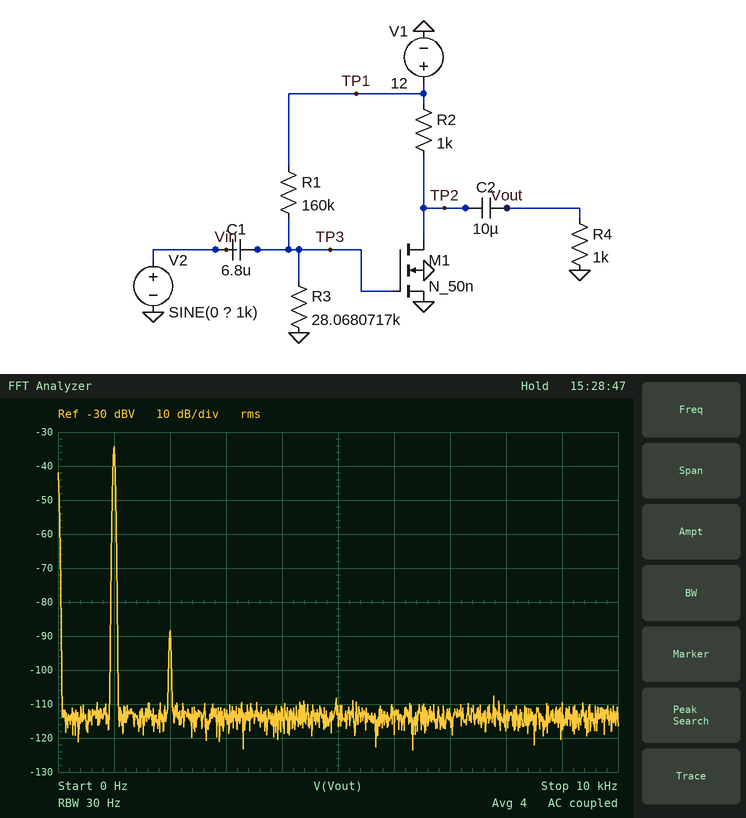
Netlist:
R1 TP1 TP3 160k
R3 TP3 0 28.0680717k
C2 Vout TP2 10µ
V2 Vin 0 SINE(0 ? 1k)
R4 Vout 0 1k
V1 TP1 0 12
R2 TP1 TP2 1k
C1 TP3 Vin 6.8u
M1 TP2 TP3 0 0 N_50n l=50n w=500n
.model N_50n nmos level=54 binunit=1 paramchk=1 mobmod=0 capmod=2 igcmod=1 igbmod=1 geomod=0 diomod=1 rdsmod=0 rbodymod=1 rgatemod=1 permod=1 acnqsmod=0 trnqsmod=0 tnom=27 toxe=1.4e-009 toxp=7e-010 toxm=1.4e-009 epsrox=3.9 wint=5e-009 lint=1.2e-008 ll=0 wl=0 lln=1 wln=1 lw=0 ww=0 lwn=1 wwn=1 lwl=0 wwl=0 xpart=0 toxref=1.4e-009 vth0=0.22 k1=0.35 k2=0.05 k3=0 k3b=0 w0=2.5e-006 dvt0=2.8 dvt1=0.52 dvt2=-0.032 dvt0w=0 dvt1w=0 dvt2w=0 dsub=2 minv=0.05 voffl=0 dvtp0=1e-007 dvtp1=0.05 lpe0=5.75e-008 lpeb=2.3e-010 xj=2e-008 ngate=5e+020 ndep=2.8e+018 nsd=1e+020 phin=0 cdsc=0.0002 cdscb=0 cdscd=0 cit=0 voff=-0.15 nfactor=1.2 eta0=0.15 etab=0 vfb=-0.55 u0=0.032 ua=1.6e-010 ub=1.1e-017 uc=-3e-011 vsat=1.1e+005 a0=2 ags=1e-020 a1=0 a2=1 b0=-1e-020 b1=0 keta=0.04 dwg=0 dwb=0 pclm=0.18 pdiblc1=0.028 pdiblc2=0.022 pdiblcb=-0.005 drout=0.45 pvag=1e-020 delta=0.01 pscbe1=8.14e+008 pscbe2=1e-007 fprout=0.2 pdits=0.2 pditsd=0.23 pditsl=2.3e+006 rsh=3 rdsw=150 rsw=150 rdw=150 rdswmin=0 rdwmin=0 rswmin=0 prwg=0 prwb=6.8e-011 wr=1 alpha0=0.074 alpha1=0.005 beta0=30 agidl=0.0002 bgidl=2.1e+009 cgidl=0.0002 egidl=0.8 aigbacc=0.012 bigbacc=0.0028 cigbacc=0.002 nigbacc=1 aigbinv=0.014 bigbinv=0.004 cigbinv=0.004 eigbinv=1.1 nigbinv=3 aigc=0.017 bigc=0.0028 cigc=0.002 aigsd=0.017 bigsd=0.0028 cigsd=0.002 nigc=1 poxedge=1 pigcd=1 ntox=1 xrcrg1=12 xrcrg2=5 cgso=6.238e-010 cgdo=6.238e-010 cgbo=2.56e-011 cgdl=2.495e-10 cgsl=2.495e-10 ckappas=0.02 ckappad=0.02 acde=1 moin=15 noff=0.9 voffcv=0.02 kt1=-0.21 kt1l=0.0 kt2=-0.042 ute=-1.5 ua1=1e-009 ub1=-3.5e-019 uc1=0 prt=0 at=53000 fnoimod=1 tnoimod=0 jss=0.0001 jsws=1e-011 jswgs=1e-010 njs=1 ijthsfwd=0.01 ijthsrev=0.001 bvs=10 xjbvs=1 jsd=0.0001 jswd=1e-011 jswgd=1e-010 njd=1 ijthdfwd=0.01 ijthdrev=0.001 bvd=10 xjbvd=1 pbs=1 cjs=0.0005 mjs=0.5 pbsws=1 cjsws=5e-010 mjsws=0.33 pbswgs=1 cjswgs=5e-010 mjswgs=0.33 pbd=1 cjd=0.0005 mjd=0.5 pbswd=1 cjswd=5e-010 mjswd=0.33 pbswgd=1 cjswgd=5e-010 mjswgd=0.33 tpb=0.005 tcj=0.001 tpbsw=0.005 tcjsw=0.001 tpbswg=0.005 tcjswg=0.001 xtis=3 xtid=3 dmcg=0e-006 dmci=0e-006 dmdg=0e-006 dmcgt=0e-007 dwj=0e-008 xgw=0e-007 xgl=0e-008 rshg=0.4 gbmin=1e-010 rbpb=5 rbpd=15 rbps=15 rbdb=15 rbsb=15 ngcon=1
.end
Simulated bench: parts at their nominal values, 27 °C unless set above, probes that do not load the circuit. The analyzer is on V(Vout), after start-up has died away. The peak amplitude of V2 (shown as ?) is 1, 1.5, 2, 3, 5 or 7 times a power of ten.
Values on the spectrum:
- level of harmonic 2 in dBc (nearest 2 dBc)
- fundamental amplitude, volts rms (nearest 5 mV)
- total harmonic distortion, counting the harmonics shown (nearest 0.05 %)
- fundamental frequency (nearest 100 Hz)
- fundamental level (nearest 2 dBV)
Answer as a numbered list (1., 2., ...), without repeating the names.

1. -54 dBc
2. 20 mV
3. 0.20 %
4. 1.0 kHz
5. -34 dBV
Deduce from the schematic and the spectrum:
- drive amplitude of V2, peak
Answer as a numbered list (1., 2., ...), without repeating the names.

1. 50 mV
